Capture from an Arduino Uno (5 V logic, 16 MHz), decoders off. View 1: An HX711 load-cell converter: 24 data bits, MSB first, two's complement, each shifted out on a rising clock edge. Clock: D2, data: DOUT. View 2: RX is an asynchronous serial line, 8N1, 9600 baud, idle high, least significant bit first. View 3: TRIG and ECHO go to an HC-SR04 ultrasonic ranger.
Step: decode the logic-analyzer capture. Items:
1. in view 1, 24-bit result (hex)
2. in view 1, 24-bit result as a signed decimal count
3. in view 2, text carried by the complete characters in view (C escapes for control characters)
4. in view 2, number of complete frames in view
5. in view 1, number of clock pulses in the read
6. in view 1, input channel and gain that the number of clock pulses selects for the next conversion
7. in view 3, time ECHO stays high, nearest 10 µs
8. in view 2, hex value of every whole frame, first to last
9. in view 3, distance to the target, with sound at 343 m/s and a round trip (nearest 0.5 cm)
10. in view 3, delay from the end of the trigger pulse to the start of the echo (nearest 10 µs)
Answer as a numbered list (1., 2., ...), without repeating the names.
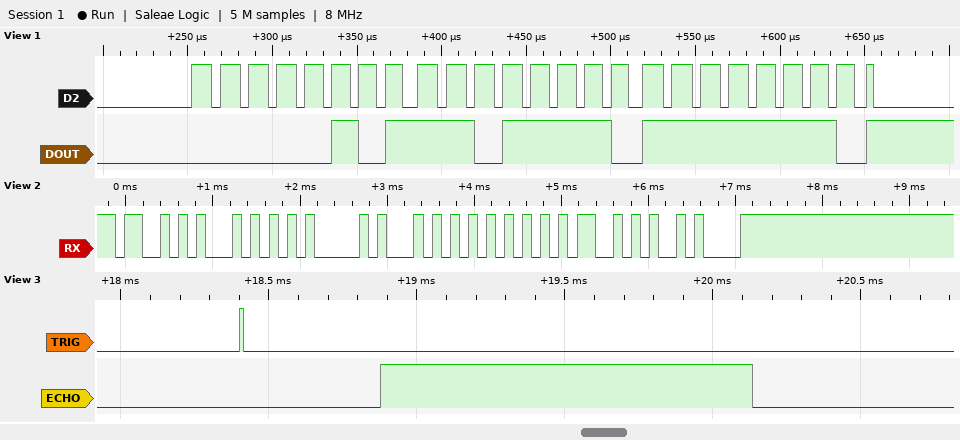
1. 0x05DEFE
2. 384766
3. "STATUS\n"
4. 7
5. 25
6. channel A, gain 128
7. 1260 µs
8. 53 54 41 54 55 53 0A
9. 21.5 cm
10. 460 µs
